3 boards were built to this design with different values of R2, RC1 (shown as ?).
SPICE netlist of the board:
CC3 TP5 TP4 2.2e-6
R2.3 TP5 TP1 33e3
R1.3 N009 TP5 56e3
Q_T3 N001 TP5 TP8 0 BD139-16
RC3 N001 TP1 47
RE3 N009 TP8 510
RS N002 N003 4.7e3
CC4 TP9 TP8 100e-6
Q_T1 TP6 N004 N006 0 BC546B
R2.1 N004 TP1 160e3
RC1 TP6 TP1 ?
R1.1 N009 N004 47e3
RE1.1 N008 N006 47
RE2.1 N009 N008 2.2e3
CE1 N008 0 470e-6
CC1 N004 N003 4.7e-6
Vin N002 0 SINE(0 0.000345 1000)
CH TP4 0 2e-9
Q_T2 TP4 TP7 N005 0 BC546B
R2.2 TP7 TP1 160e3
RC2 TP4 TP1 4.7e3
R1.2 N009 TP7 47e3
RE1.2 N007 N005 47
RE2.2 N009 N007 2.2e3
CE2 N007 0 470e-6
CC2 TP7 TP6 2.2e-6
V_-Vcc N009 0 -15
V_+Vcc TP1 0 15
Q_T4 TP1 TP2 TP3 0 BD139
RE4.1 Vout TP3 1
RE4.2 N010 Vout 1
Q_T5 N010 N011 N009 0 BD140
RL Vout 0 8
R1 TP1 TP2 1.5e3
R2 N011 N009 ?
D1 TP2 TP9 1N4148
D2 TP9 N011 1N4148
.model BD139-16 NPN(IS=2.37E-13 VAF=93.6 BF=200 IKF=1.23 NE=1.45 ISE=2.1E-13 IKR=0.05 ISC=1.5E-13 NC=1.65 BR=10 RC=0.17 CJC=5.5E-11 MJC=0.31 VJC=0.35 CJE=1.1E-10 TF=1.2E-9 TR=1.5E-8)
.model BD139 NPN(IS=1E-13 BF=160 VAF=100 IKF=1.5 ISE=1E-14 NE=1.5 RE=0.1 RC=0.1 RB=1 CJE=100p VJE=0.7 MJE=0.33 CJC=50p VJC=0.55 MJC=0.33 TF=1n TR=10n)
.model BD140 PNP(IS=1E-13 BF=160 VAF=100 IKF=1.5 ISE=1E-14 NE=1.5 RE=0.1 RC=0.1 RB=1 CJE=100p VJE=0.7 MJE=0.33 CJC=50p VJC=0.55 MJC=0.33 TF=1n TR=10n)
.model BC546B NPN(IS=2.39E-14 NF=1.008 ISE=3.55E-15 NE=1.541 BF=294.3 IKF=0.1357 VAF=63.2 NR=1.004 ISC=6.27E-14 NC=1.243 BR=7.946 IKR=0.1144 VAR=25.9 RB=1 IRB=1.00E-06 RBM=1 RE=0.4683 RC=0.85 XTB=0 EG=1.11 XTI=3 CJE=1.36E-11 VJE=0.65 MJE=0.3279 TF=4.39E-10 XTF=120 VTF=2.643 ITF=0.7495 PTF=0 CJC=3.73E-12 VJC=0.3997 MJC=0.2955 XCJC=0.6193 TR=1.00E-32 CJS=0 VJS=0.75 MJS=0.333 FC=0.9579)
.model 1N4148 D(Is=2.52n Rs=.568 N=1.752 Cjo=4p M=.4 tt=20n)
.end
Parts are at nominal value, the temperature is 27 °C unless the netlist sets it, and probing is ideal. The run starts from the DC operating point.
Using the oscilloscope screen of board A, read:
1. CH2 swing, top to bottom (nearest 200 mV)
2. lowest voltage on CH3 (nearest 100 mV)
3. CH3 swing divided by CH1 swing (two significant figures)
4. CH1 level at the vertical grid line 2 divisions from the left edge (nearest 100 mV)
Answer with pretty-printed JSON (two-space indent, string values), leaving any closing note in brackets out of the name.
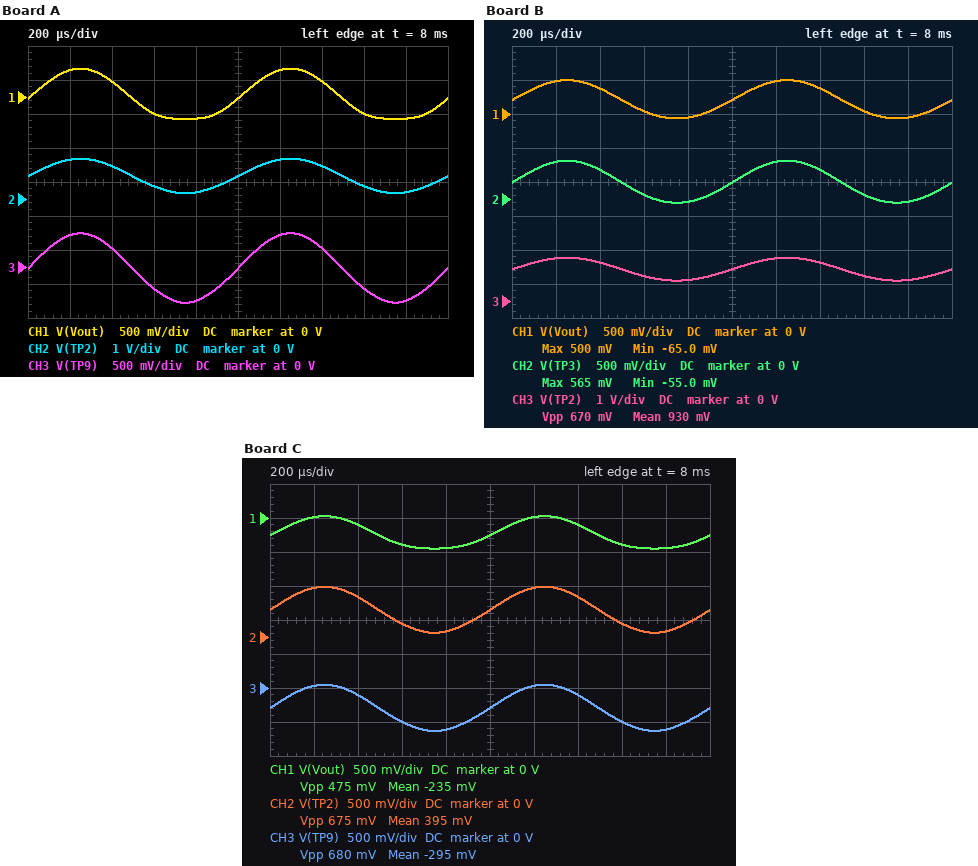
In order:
{
  "CH2 swing, top to bottom": "1.0 V",
  "lowest voltage on CH3": "-500 mV",
  "CH3 swing divided by CH1 swing": "1.4",
  "CH1 level at the vertical grid line 2 divisions from the left edge": "200 mV"
}
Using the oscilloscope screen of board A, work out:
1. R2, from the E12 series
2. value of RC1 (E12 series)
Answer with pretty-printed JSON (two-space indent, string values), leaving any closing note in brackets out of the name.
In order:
{
  "R2, from the E12 series": "680 Ω",
  "value of RC1": "3.3 kΩ"
}
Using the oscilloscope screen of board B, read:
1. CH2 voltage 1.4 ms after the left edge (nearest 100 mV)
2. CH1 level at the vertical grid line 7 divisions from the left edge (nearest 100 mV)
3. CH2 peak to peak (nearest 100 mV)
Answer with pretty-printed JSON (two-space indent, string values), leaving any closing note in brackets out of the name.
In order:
{
  "CH2 voltage 1.4 ms after the left edge": "400 mV",
  "CH1 level at the vertical grid line 7 divisions from the left edge": "400 mV",
  "CH2 peak to peak": "600 mV"
}
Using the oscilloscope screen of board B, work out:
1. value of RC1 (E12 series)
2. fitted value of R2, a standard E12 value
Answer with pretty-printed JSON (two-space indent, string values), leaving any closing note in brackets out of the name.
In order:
{
  "value of RC1": "1.8 kΩ",
  "fitted value of R2, a standard E12 value": "1 kΩ"
}
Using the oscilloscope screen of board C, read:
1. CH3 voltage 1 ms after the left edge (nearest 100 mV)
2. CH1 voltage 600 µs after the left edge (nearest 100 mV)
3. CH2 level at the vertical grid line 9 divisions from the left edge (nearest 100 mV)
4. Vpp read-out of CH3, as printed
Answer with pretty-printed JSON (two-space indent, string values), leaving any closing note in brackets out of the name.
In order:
{
  "CH3 voltage 1 ms after the left edge": "-300 mV",
  "CH1 voltage 600 µs after the left edge": "-400 mV",
  "CH2 level at the vertical grid line 9 divisions from the left edge": "100 mV",
  "Vpp read-out of CH3, as printed": "680 mV"
}
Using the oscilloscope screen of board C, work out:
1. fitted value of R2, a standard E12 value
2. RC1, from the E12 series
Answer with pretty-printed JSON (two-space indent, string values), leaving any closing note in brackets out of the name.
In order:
{
  "fitted value of R2, a standard E12 value": "470 Ω",
  "RC1, from the E12 series": "2.2 kΩ"
}
